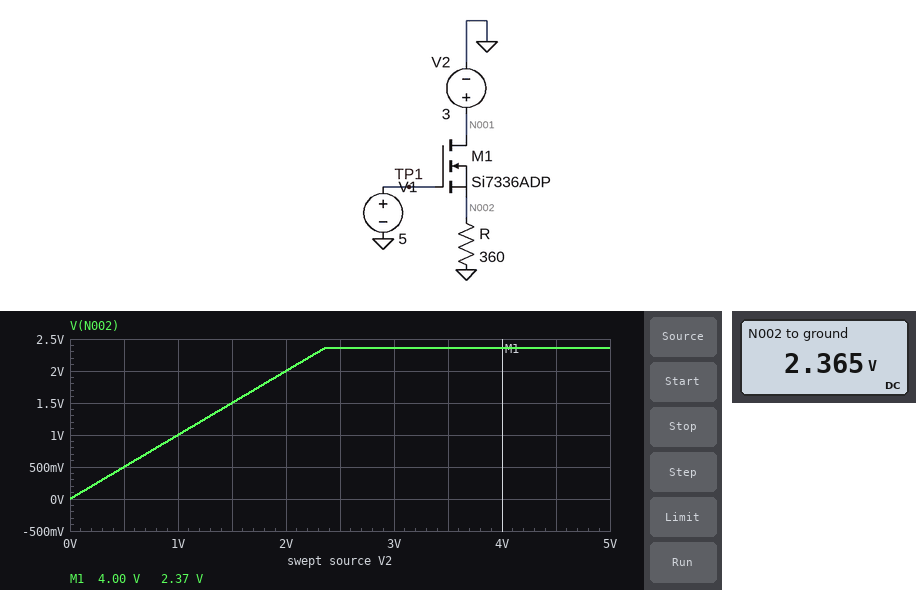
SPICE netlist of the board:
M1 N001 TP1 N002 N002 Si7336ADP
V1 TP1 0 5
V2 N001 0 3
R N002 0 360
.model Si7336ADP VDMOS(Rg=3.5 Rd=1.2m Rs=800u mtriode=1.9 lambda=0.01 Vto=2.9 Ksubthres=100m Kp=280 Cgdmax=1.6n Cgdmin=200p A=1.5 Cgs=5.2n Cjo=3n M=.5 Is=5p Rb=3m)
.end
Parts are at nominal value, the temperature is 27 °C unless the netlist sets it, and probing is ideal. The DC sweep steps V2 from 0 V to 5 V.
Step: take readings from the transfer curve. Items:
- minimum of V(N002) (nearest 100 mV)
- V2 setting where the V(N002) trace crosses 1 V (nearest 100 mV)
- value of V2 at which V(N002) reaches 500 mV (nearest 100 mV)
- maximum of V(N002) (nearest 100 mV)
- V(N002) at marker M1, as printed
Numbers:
0 V
1.0 V
500 mV
2.4 V
2.37 V
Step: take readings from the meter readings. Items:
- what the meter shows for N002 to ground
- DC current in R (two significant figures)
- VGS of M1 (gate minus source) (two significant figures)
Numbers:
2.365 V
6.6 mA
2.6 V
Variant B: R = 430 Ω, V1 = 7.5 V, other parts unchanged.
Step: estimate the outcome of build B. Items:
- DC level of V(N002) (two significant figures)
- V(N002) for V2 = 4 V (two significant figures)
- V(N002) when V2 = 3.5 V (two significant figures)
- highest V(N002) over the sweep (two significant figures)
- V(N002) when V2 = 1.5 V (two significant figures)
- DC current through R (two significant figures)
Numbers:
3.0 V
4.0 V
3.5 V
4.8 V
1.5 V
7.0 mA
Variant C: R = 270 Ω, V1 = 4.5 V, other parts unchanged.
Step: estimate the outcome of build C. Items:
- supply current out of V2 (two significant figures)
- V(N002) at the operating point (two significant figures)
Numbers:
6.9 mA
1.9 V
